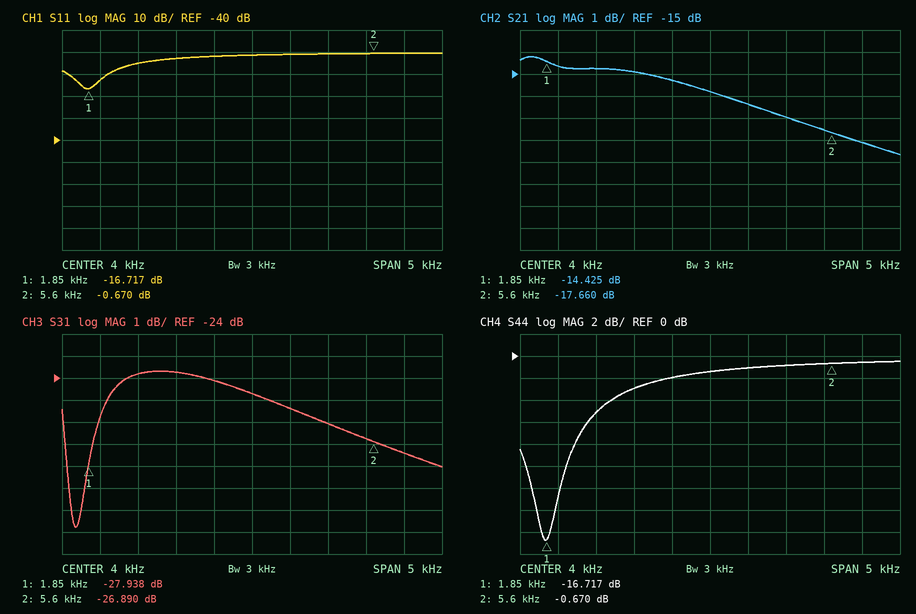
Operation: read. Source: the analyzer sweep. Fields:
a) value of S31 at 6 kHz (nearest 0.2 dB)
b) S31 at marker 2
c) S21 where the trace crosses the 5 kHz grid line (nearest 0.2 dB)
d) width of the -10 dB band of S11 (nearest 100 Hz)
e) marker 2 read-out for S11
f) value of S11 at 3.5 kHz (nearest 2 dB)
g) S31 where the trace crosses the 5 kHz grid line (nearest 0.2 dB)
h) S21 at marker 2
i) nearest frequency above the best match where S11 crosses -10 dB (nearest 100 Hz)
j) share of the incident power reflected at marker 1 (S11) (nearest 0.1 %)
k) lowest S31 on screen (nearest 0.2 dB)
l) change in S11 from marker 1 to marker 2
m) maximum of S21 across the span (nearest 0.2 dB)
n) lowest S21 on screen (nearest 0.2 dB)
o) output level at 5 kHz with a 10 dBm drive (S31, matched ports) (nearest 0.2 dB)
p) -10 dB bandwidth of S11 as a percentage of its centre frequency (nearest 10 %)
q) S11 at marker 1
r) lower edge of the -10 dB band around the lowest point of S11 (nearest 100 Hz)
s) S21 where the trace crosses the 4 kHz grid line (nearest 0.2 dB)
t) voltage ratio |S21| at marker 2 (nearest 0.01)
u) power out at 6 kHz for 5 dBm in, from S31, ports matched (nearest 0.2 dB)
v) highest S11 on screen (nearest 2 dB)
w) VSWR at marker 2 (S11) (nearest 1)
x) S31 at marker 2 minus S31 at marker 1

-27.4 dB
-26.890 dB
-17.0 dB
500 Hz
-0.670 dB
-2 dB
-26.0 dB
-17.660 dB
2.1 kHz
2.1 %
-30.8 dB
16.047 dB
-14.2 dB
-18.6 dB
-16.0 dBm
30 %
-16.717 dB
1.6 kHz
-15.8 dB
0.13
-22.4 dBm
0 dB
26
1.048 dB
